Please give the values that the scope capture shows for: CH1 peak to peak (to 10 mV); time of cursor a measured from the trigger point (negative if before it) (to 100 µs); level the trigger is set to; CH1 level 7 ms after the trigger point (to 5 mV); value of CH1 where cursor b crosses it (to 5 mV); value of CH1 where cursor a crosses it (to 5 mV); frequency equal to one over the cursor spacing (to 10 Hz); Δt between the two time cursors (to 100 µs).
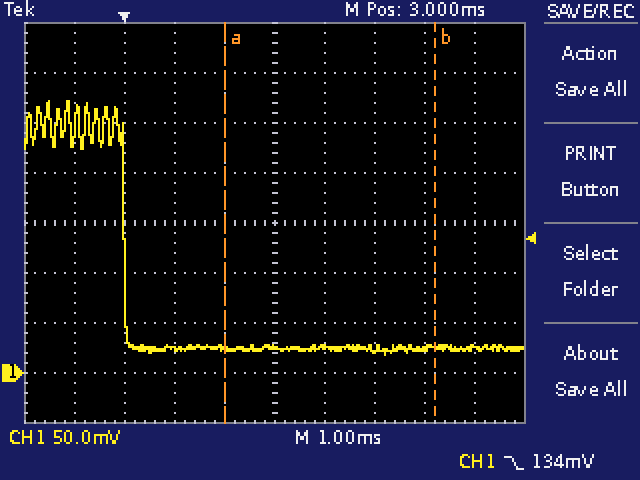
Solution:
250 mV
+2.0 ms
134 mV
25 mV
25 mV
25 mV
240 Hz
4.2 ms
